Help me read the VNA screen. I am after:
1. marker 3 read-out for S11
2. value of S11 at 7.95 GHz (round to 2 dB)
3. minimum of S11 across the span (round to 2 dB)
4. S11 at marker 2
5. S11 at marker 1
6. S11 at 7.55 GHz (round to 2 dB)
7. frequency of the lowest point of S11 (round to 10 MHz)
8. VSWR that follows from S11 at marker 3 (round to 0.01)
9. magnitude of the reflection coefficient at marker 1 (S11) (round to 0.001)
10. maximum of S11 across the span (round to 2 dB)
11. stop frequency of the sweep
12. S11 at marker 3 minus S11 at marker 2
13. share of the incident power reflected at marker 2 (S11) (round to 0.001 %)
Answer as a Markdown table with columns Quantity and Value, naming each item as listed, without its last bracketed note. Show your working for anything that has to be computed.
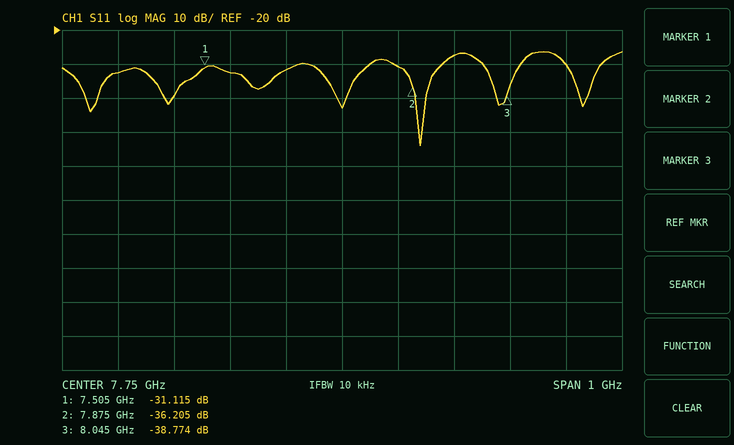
| Quantity | Value |
|---|---|
| marker 3 read-out for S11 | -38.774 dB |
| value of S11 at 7.95 GHz | -28 dB |
| minimum of S11 across the span | -54 dB |
| S11 at marker 2 | -36.205 dB |
| S11 at marker 1 | -31.115 dB |
| S11 at 7.55 GHz | -32 dB |
| frequency of the lowest point of S11 | 7.89 GHz |
| VSWR that follows from S11 at marker 3 | (1 + 0.0115)/(1 − 0.0115) ≈ 1.02 |
| magnitude of the reflection coefficient at marker 1 (S11) | 10^(-31.115/20) ≈ 0.028 |
| maximum of S11 across the span | -26 dB |
| stop frequency of the sweep | 8.25 GHz |
| S11 at marker 3 minus S11 at marker 2 | -38.774 − (-36.205) = -2.569 dB |
| share of the incident power reflected at marker 2 (S11) | 10^(-36.205/10) ≈ 0.024 % |
